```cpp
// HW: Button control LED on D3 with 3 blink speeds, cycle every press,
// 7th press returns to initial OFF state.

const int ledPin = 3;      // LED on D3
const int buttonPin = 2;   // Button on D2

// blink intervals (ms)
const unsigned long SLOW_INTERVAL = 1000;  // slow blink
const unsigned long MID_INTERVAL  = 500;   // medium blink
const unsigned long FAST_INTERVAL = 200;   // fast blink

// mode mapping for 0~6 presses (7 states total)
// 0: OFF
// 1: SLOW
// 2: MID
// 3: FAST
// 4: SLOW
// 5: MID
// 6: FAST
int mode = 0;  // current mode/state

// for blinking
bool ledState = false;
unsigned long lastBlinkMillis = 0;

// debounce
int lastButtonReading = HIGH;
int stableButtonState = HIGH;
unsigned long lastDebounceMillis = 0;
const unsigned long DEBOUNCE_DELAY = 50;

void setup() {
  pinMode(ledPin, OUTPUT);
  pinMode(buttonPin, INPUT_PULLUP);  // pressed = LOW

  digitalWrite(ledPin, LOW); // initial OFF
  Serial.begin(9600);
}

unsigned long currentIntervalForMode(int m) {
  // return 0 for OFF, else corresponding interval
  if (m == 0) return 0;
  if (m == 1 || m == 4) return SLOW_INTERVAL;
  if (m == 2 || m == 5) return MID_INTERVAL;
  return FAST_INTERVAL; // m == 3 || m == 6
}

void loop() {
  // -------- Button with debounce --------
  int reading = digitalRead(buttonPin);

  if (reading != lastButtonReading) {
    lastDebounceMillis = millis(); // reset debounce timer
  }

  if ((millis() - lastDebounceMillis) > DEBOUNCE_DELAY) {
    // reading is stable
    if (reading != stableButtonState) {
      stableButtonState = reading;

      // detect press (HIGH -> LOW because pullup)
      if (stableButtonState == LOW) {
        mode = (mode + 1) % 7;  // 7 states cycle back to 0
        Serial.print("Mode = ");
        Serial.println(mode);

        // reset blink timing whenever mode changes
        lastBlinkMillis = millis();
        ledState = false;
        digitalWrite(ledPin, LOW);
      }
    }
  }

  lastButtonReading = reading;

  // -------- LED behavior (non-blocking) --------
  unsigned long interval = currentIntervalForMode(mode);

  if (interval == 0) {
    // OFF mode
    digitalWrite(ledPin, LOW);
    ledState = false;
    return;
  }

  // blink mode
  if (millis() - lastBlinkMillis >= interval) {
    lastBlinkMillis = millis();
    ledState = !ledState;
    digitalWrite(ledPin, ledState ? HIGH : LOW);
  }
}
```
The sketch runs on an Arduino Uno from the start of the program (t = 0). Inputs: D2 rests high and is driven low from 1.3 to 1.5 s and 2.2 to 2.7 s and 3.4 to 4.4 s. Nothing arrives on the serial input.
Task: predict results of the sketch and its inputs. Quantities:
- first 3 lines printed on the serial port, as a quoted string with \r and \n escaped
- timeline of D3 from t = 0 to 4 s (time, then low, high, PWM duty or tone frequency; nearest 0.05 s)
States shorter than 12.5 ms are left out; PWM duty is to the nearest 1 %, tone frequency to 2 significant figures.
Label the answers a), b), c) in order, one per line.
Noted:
a) "Mode = 1\r\nMode = 2\r\nMode = 3\r\n"
b) 0 s low; 2.75 s high; 3.25 s low; 3.65 s high; 3.85 s low
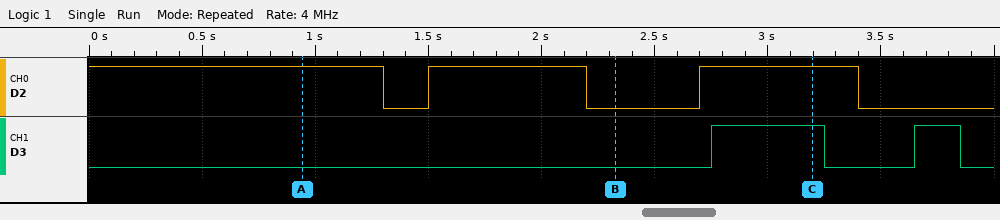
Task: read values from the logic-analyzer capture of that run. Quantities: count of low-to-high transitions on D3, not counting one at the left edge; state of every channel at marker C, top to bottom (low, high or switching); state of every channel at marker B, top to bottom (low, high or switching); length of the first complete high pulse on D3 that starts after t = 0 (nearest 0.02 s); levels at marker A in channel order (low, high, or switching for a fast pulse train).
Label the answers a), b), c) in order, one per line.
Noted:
a) 2
b) D2 high, D3 high
c) D2 low, D3 low
d) 0.50 s
e) D2 high, D3 low
